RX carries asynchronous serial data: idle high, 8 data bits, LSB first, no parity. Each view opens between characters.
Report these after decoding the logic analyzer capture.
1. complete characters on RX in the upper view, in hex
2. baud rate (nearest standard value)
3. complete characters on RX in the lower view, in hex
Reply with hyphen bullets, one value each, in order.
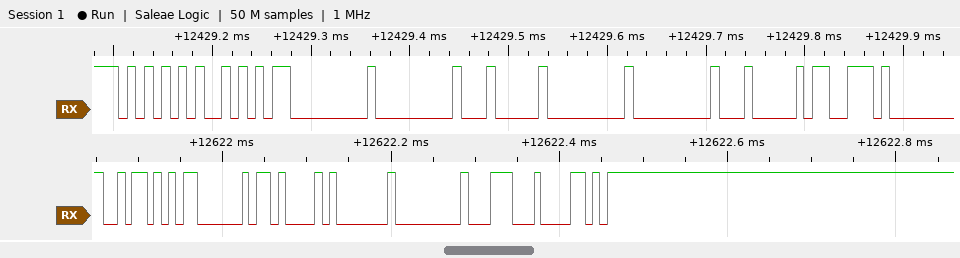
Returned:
- 55, AA, 00, 00, 04, 00, 00, 04, 73
- 115200 baud
- 5A, 03, 0B, 01, 00, 1C, 58
